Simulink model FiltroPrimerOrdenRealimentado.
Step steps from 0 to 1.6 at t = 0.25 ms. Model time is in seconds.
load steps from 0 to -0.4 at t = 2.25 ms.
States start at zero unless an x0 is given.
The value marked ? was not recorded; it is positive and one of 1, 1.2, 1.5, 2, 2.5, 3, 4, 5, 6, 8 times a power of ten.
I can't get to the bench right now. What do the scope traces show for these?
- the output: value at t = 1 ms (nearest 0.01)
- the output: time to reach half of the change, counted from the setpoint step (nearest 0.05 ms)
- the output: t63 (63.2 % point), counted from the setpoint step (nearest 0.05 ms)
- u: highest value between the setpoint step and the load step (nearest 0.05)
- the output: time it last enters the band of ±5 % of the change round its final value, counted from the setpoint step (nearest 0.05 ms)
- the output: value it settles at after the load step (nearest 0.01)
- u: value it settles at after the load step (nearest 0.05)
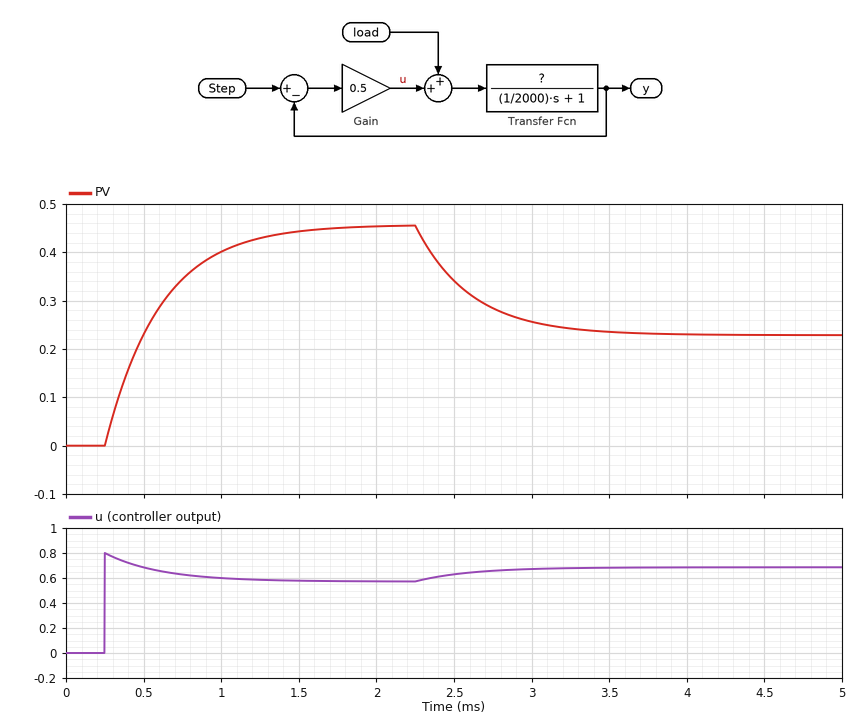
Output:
0.40
0.25 ms
0.35 ms
0.80
1.05 ms
0.23
0.70
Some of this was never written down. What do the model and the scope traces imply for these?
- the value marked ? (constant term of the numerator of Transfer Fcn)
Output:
0.8
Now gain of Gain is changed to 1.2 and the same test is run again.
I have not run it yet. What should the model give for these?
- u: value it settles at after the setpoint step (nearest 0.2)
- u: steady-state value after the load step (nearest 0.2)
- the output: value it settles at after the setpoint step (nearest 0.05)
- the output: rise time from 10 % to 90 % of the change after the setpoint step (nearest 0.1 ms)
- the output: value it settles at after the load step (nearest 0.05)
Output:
1.0
1.2
0.80
0.6 ms
0.60
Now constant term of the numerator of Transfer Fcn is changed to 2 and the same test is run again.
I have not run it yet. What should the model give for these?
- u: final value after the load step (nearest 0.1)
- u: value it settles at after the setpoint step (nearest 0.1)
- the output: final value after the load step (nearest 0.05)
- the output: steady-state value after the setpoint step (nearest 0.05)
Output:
0.6
0.4
0.40
0.80
